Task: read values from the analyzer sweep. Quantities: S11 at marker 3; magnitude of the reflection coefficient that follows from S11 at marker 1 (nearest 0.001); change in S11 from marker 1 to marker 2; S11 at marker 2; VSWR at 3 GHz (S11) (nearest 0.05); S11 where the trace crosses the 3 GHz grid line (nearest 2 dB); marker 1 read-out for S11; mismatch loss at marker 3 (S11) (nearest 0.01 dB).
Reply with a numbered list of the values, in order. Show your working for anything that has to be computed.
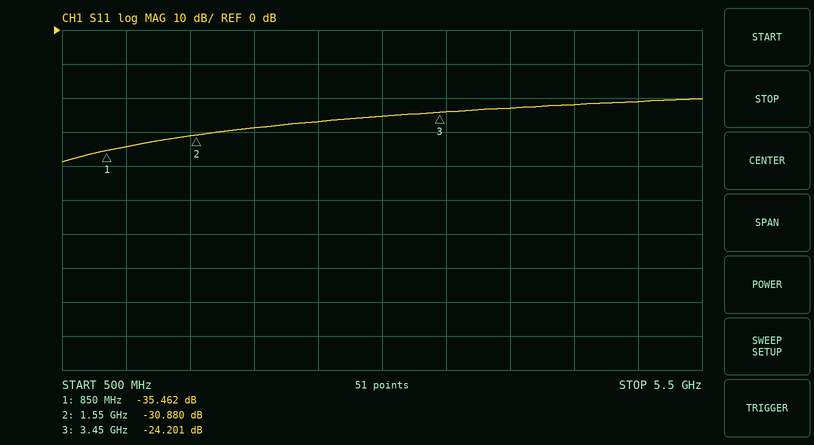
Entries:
1. -24.201 dB
2. 10^(-35.462/20) ≈ 0.017
3. -30.88 − (-35.462) = 4.582 dB
4. -30.880 dB
5. |Γ| = 10^(-26/20) = 0.0501; VSWR = (1 + 0.0501)/(1 − 0.0501) ≈ 1.11, so 1.10 to the nearest 0.05
6. -26 dB
7. -35.462 dB
8. −10 log10(1 − 10^(-24.201/10)) ≈ 0.02 dB
